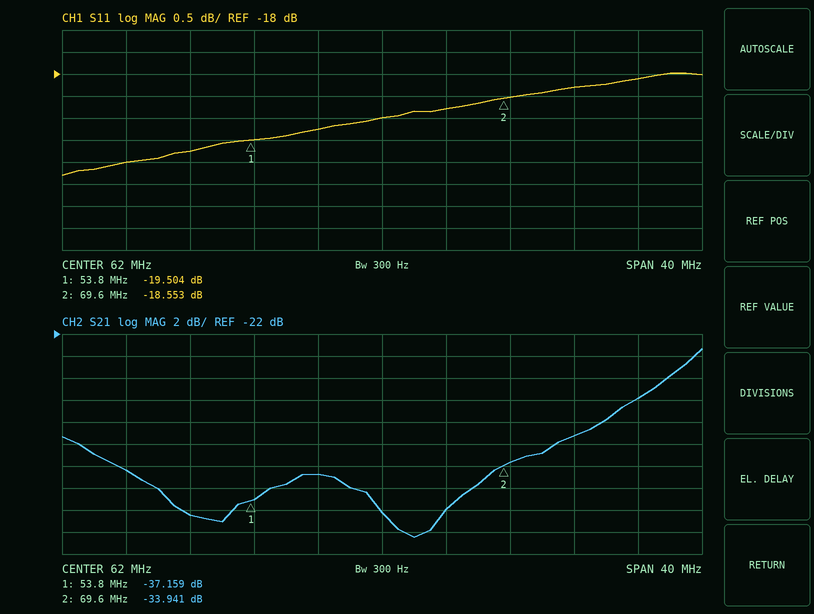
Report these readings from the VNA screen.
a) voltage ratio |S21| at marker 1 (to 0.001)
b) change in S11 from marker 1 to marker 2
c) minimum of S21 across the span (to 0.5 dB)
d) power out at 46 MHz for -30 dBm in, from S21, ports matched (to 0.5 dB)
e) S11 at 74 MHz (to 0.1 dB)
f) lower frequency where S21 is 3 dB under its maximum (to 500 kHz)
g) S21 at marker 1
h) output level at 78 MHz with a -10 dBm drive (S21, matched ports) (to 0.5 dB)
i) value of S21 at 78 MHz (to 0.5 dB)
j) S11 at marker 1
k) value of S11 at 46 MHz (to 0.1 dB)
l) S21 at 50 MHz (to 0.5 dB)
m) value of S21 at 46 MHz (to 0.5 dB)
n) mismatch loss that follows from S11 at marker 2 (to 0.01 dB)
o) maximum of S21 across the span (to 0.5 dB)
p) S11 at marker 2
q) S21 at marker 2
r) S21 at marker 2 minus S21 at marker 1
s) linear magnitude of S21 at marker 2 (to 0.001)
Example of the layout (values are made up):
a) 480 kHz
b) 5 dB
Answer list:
a) 0.014
b) 0.951 dB
c) -40.5 dB
d) -64.5 dBm
e) -18.3 dB
f) 79.5 MHz
g) -37.159 dB
h) -38.0 dBm
i) -28.0 dB
j) -19.504 dB
k) -20.0 dB
l) -38.5 dB
m) -34.5 dB
n) 0.06 dB
o) -23.5 dB
p) -18.553 dB
q) -33.941 dB
r) 3.218 dB
s) 0.020
